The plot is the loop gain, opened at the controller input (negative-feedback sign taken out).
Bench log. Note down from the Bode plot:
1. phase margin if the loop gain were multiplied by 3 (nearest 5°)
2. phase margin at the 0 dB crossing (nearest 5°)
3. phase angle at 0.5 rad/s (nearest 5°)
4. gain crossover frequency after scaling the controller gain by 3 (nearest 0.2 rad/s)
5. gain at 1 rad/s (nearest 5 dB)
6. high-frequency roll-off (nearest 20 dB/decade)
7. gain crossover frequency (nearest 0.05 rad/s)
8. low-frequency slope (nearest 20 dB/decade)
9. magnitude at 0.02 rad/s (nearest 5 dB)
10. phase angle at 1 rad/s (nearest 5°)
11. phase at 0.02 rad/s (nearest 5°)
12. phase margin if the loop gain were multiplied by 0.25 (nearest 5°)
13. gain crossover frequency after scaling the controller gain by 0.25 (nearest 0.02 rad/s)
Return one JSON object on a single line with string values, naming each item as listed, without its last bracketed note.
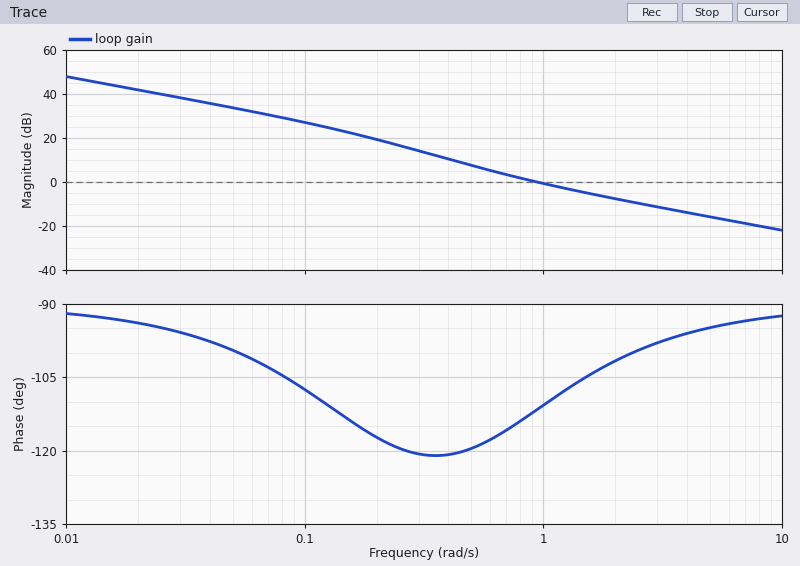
{"phase margin if the loop gain were multiplied by 3": "80°", "phase margin at the 0 dB crossing": "70°", "phase angle at 0.5 rad/s": "-120°", "gain crossover frequency after scaling the controller gain by 3": "2.4 rad/s", "gain at 1 rad/s": "0 dB", "high-frequency roll-off": "-20 dB/decade", "gain crossover frequency": "0.95 rad/s", "low-frequency slope": "-20 dB/decade", "magnitude at 0.02 rad/s": "40 dB", "phase angle at 1 rad/s": "-110°", "phase at 0.02 rad/s": "-95°", "phase margin if the loop gain were multiplied by 0.25": "60°", "gain crossover frequency after scaling the controller gain by 0.25": "0.36 rad/s"}
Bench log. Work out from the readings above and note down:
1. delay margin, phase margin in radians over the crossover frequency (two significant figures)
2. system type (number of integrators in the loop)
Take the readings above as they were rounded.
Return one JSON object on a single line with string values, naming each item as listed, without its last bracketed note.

{"delay margin, phase margin in radians over the crossover frequency": "1.3 s", "system type": "1"}
